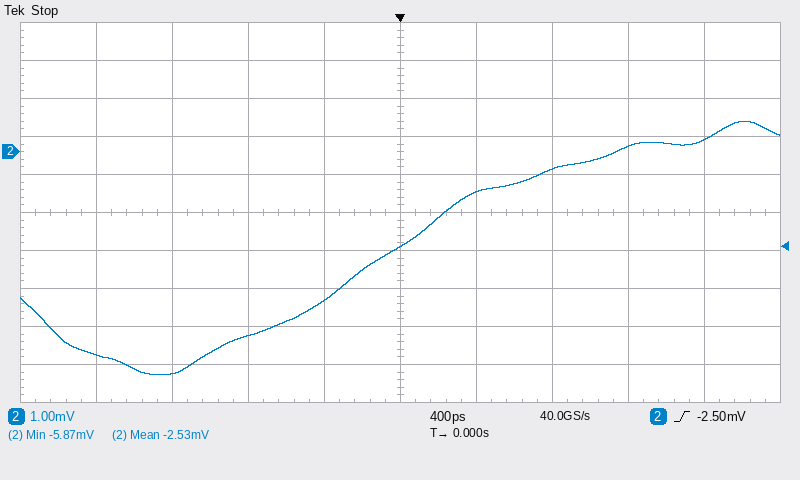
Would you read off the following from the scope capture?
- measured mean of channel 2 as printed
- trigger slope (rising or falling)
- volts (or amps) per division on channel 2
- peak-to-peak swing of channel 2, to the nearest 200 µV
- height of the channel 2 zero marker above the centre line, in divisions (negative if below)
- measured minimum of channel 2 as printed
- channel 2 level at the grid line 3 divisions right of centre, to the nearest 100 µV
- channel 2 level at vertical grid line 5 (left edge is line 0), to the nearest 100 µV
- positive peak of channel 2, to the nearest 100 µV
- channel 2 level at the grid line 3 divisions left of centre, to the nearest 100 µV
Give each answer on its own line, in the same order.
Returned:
-2.53 mV
rising
1 mV
6.6 mV
+1.6 div
-5.87 mV
100 µV
-2.5 mV
800 µV
-5.8 mV
